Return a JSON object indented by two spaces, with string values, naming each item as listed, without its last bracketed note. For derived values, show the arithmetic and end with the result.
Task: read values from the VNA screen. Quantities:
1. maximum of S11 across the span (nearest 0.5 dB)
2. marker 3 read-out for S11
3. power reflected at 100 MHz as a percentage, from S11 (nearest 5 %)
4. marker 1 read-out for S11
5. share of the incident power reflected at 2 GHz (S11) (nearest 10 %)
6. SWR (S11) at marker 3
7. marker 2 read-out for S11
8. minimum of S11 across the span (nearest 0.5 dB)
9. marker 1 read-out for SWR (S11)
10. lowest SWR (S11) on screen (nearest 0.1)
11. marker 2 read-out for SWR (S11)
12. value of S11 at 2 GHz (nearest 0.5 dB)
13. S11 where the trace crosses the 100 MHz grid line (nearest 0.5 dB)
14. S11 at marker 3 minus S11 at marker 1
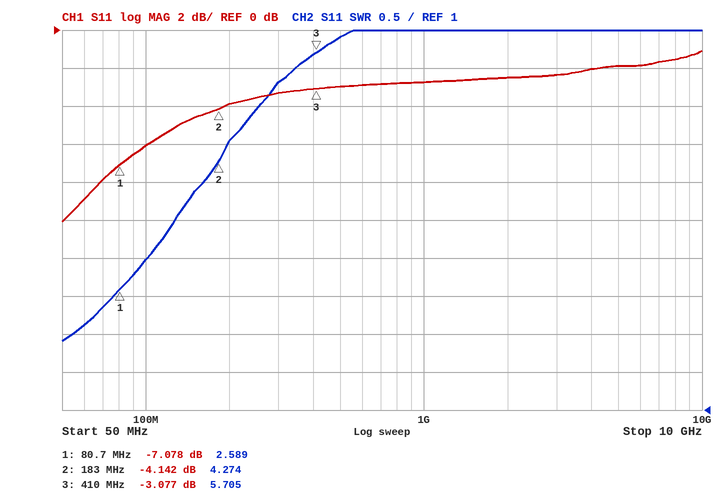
{
  "maximum of S11 across the span": "-1.0 dB",
  "marker 3 read-out for S11": "-3.077 dB",
  "power reflected at 100 MHz as a percentage, from S11": "10^(-6/10) ≈ 25 %",
  "marker 1 read-out for S11": "-7.078 dB",
  "share of the incident power reflected at 2 GHz (S11)": "10^(-2.5/10) ≈ 56.2 %, so 60 % to the nearest 10 %",
  "SWR (S11) at marker 3": "5.705",
  "marker 2 read-out for S11": "-4.142 dB",
  "minimum of S11 across the span": "-10.0 dB",
  "marker 1 read-out for SWR": "2.589",
  "lowest SWR (S11) on screen": "1.9",
  "marker 2 read-out for SWR": "4.274",
  "value of S11 at 2 GHz": "-2.5 dB",
  "S11 where the trace crosses the 100 MHz grid line": "-6.0 dB",
  "S11 at marker 3 minus S11 at marker 1": "-3.077 − (-7.078) = 4.001 dB"
}
